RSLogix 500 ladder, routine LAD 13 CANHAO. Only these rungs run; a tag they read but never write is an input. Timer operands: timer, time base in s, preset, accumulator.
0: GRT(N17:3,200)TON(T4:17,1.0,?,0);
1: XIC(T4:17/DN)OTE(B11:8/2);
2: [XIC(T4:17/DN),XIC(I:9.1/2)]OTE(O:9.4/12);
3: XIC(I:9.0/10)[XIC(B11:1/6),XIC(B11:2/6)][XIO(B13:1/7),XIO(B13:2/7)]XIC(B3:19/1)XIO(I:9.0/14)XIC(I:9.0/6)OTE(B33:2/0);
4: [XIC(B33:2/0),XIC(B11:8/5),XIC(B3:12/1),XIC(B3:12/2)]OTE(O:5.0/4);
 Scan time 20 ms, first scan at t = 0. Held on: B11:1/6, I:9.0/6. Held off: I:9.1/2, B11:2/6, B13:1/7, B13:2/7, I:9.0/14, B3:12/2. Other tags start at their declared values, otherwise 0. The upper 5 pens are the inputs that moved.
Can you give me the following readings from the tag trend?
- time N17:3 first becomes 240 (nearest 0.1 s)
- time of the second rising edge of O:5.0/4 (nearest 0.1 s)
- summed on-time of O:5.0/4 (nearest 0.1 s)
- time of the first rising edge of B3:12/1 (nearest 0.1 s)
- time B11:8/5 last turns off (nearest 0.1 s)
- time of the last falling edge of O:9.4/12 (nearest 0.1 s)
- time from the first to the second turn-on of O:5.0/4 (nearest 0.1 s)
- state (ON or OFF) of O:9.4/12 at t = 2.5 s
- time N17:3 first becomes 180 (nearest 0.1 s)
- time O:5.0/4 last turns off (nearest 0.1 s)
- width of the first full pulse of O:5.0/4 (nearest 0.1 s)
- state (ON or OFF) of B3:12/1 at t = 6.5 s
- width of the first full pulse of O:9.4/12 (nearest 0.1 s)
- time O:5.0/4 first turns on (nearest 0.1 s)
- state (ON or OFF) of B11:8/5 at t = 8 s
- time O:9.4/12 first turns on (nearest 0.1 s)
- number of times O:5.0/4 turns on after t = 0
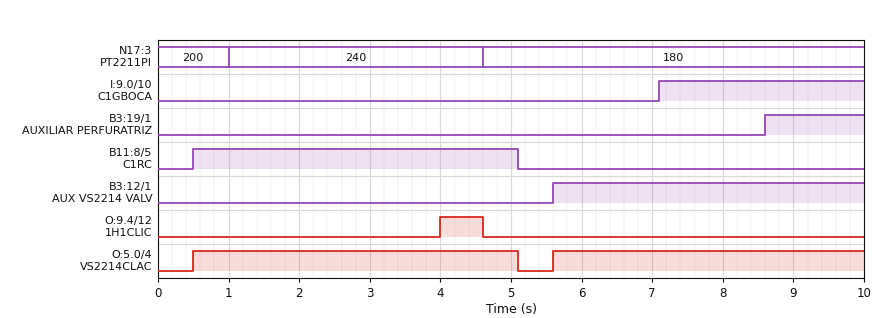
1.0 s
5.6 s
9.0 s
5.6 s
5.1 s
4.6 s
5.1 s
OFF
4.6 s
5.1 s
4.6 s
ON
0.6 s
0.5 s
OFF
4.0 s
2
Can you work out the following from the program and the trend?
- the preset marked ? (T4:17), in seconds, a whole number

3 s
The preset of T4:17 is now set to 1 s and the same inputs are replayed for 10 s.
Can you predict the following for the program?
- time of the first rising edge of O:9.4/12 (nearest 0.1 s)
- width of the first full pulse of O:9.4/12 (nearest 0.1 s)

2.0 s
2.6 s
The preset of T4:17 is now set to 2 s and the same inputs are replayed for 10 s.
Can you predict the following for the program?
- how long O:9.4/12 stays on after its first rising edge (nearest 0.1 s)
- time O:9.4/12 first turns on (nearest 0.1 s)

1.6 s
3.0 s
